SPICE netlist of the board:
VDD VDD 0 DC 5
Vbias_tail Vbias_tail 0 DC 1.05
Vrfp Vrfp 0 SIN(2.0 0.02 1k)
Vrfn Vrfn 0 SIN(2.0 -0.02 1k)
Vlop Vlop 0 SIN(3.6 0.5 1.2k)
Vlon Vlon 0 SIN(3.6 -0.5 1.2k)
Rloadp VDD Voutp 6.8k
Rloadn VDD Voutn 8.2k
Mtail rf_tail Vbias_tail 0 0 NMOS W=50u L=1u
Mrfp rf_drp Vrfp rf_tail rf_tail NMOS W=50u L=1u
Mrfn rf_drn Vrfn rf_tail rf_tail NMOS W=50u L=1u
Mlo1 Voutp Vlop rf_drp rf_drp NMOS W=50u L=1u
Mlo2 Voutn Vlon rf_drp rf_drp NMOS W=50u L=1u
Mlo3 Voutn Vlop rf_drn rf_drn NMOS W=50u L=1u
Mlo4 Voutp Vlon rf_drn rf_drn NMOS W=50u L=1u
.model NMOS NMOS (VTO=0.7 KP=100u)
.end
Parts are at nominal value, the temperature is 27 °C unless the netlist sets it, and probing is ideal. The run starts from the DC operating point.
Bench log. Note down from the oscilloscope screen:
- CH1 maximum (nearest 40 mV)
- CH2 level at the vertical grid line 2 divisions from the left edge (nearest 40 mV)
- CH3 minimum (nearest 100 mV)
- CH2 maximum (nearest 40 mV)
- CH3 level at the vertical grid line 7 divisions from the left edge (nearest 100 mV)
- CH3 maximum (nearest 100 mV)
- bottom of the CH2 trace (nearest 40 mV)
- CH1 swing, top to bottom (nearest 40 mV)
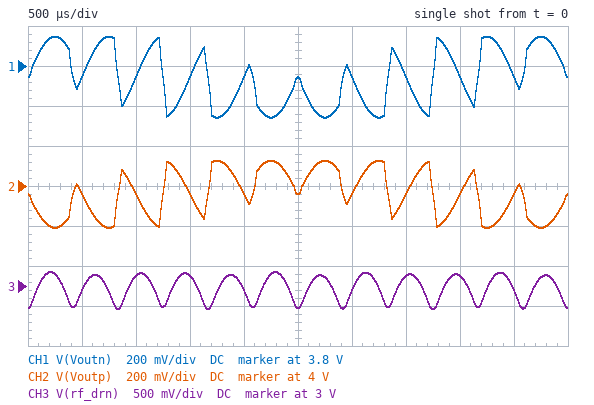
3.96 V
3.96 V
2.7 V
4.12 V
3.1 V
3.2 V
3.80 V
400 mV
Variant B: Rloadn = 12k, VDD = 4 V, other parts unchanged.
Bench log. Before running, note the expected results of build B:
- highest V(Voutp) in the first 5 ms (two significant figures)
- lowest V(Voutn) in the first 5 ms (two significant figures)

2.9 V
2.3 V
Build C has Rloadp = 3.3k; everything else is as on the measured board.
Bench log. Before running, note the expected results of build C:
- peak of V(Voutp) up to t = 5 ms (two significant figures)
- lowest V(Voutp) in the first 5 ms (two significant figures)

4.6 V
4.4 V
